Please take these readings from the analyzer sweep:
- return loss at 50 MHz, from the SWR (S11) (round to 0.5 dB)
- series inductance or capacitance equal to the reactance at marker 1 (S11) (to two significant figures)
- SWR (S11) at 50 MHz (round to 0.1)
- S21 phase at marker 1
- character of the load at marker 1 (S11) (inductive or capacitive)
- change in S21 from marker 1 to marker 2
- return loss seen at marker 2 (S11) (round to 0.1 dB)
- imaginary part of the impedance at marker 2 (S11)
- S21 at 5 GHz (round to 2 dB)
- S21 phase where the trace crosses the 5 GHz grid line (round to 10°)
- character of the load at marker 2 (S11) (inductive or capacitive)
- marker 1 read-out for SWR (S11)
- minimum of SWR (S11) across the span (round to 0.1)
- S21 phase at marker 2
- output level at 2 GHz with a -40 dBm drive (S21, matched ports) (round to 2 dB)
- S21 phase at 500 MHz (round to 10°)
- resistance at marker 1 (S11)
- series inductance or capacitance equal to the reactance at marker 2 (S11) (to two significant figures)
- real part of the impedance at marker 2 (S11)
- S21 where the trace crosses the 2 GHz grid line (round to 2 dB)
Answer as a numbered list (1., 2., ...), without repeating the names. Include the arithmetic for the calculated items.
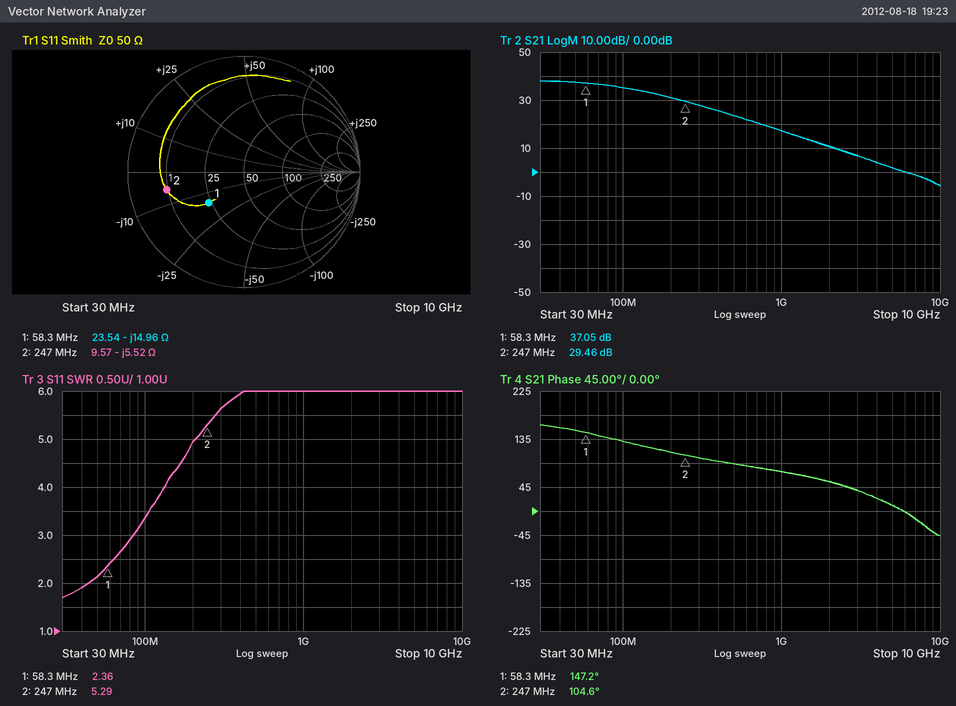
1. −20 log10((2.1 − 1)/(2.1 + 1)) ≈ 9.0 dB
2. C = 1/(2π × 58.3 MHz × 14.96 Ω) ≈ 182 pF, so 180 pF to two significant figures
3. 2.1
4. 147.2°
5. capacitive
6. 29.46 − (37.05) = -7.59 dB
7. 3.3 dB
8. -5.52 Ω
9. 2 dB
10. 10°
11. capacitive
12. 2.36
13. 1.7
14. 104.6°
15. -40 dBm + (10 dB) = -30 dBm
16. 90°
17. 23.54 Ω
18. C = 1/(2π × 247 MHz × 5.52 Ω) ≈ 117 pF, so 120 pF to two significant figures
19. 9.57 Ω
20. 10 dB
